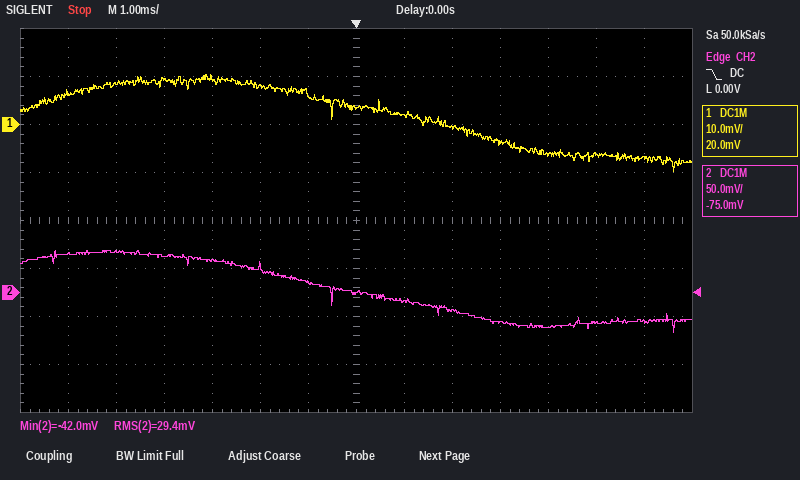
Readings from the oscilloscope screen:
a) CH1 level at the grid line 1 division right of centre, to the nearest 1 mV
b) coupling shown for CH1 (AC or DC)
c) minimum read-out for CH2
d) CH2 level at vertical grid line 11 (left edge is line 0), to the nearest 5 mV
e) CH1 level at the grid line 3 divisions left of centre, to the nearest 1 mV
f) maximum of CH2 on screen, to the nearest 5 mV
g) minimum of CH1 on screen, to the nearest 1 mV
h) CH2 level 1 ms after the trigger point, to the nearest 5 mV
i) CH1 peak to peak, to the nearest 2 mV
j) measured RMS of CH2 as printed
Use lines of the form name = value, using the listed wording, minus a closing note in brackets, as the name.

CH1 level at the grid line 1 division right of centre, to the nearest 1 mV = 2 mV
coupling shown for CH1 = DC
minimum read-out for CH2 = -42.0 mV
CH2 level at vertical grid line 11 (left edge is line 0), to the nearest 5 mV = -35 mV
CH1 level at the grid line 3 divisions left of centre, to the nearest 1 mV = 10 mV
maximum of CH2 on screen, to the nearest 5 mV = 45 mV
minimum of CH1 on screen, to the nearest 1 mV = -10 mV
CH2 level 1 ms after the trigger point, to the nearest 5 mV = -10 mV
CH1 peak to peak, to the nearest 2 mV = 20 mV
measured RMS of CH2 as printed = 29.4 mV
